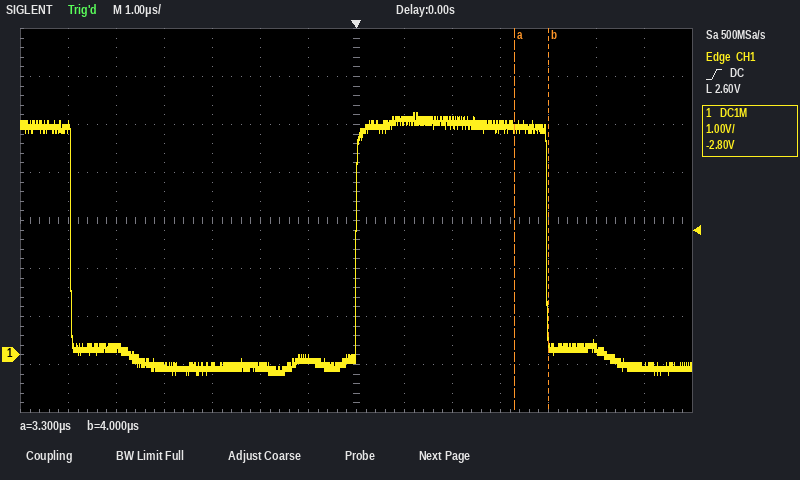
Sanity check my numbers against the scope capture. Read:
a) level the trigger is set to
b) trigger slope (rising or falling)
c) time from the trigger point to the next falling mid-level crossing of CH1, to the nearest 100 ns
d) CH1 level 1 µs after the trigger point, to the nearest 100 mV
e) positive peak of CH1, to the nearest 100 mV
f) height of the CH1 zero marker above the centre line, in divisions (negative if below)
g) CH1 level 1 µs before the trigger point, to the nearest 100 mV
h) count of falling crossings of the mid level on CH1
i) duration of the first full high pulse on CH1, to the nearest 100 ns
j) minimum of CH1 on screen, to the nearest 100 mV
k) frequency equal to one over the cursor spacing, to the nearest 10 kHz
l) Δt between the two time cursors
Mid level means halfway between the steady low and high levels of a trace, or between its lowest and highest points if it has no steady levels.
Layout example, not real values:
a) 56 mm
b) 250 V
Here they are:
a) 2.60 V
b) rising
c) 4.0 µs
d) 4.9 V
e) 5.0 V
f) -2.8 div
g) -100 mV
h) 2
i) 4.0 µs
j) -400 mV
k) 1.43 MHz
l) 700 ns
